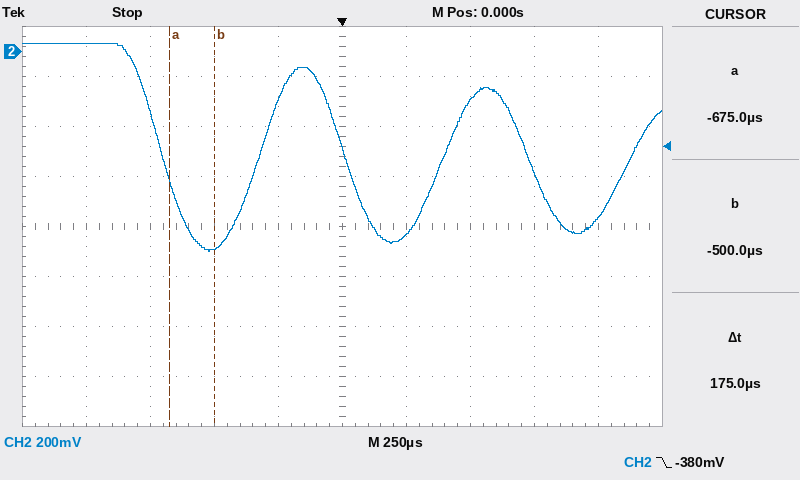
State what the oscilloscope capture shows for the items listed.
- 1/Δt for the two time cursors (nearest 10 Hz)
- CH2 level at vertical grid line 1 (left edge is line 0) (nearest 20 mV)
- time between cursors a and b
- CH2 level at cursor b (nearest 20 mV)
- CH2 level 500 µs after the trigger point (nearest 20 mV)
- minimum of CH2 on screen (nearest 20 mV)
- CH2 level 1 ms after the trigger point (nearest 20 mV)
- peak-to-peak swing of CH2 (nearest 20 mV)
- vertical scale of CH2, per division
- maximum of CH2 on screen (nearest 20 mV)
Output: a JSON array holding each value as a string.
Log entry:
["5.71 kHz", "40 mV", "175 µs", "-780 mV", "-200 mV", "-800 mV", "-660 mV", "840 mV", "200 mV", "40 mV"]
